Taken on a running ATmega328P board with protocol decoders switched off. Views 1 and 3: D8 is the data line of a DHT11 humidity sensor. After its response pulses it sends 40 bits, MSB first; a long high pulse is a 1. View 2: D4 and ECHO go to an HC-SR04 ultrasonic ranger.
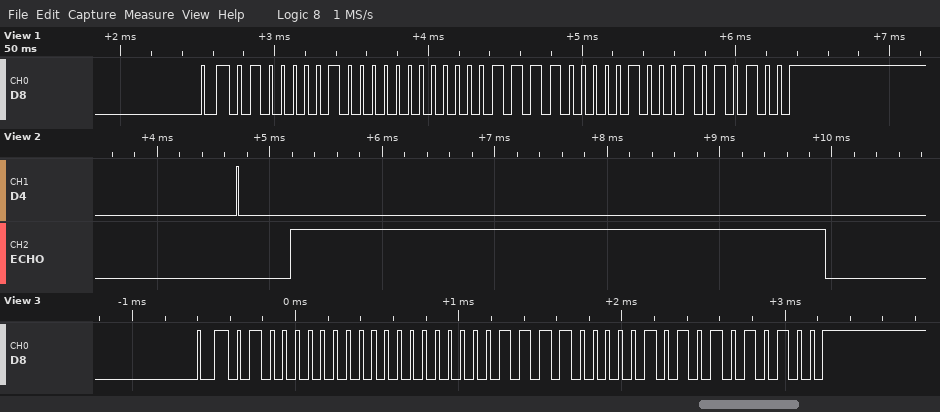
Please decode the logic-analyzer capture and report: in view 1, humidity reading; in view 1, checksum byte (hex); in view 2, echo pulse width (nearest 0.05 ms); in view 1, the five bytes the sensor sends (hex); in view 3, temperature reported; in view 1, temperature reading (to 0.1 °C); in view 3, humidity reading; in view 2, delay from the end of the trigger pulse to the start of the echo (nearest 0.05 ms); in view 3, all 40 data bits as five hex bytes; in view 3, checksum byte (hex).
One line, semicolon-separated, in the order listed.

65 %; 0x54; 4.75 ms; 41 00 0F 04 54; 15.5 °C; 15.4 °C; 64 %; 0.45 ms; 40 00 0F 05 54; 0x54
